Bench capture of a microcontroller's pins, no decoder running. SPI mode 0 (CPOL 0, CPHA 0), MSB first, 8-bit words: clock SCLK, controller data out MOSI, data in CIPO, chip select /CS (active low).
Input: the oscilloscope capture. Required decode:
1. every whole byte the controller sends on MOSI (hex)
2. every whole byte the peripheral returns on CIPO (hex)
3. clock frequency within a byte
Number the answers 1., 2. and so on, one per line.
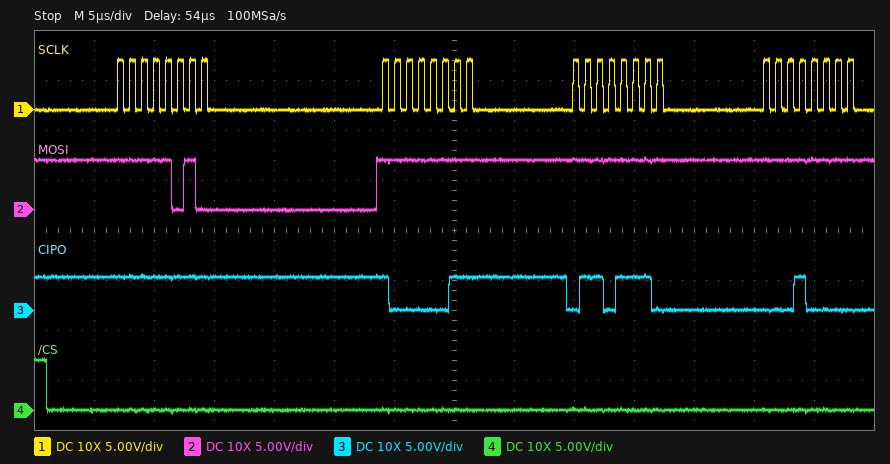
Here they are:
1. 0xFA 0xFF 0xFF 0xFF
2. 0xFF 0x83 0x6E 0x10
3. 1 MHz
